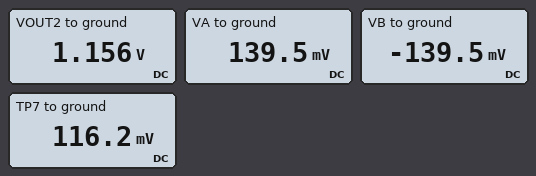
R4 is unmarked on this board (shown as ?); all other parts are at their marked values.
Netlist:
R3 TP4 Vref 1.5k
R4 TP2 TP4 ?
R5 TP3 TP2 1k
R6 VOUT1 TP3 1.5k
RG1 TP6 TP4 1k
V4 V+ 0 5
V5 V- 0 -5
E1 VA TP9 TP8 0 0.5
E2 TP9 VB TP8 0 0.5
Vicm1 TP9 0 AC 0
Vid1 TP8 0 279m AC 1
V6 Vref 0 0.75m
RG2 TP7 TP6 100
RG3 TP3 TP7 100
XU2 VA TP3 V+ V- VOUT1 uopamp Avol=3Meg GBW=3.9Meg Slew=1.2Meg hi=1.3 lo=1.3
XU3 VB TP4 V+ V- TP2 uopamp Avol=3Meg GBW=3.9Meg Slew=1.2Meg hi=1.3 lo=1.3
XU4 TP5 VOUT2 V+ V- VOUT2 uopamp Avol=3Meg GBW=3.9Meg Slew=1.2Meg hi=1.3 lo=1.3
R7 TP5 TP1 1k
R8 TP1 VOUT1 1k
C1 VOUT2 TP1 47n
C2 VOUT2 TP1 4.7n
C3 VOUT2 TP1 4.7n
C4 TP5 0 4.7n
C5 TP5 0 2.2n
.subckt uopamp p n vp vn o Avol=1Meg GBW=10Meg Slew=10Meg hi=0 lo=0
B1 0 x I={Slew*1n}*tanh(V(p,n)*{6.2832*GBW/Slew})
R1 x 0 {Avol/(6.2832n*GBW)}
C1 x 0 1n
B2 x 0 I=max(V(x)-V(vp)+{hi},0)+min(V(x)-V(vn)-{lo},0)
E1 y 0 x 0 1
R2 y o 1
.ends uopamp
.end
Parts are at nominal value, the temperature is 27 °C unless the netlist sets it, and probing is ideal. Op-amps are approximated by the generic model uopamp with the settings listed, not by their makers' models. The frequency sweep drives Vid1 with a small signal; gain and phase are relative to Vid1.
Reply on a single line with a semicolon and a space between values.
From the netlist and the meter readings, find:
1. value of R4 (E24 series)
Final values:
510 Ω
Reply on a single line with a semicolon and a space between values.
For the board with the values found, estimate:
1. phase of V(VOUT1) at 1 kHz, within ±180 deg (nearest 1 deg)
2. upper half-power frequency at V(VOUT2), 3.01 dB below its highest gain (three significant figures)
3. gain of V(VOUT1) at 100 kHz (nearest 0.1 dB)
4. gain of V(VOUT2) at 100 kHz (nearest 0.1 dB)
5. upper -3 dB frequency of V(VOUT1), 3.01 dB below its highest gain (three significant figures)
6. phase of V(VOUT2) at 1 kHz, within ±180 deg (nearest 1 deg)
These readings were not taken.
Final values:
0 deg; 9.55 kHz; 12.3 dB; -31.5 dB; 763 kHz; -5 deg
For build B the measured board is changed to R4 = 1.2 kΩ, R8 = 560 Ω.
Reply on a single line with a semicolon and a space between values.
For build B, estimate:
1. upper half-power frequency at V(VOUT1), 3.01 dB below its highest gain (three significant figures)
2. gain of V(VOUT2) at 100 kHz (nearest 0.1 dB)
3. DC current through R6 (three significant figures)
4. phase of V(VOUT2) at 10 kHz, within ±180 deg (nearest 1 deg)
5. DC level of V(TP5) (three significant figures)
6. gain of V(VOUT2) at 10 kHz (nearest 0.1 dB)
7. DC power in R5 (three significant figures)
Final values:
570 kHz; -24.2 dB; 903 µA; -80 deg; 1.49 V; 17.8 dB; 449 µW
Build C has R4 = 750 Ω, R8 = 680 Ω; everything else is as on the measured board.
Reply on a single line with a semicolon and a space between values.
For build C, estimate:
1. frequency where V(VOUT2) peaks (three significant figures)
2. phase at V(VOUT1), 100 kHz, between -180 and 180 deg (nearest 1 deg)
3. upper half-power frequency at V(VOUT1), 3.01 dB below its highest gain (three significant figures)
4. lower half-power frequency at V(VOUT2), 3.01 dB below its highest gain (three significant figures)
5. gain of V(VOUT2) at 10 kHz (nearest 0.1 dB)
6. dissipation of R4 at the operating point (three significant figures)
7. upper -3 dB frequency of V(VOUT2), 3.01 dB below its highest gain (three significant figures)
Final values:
8.43 kHz; -9 deg; 684 kHz; 2.82 kHz; 15.9 dB; 79.7 µW; 11.6 kHz
